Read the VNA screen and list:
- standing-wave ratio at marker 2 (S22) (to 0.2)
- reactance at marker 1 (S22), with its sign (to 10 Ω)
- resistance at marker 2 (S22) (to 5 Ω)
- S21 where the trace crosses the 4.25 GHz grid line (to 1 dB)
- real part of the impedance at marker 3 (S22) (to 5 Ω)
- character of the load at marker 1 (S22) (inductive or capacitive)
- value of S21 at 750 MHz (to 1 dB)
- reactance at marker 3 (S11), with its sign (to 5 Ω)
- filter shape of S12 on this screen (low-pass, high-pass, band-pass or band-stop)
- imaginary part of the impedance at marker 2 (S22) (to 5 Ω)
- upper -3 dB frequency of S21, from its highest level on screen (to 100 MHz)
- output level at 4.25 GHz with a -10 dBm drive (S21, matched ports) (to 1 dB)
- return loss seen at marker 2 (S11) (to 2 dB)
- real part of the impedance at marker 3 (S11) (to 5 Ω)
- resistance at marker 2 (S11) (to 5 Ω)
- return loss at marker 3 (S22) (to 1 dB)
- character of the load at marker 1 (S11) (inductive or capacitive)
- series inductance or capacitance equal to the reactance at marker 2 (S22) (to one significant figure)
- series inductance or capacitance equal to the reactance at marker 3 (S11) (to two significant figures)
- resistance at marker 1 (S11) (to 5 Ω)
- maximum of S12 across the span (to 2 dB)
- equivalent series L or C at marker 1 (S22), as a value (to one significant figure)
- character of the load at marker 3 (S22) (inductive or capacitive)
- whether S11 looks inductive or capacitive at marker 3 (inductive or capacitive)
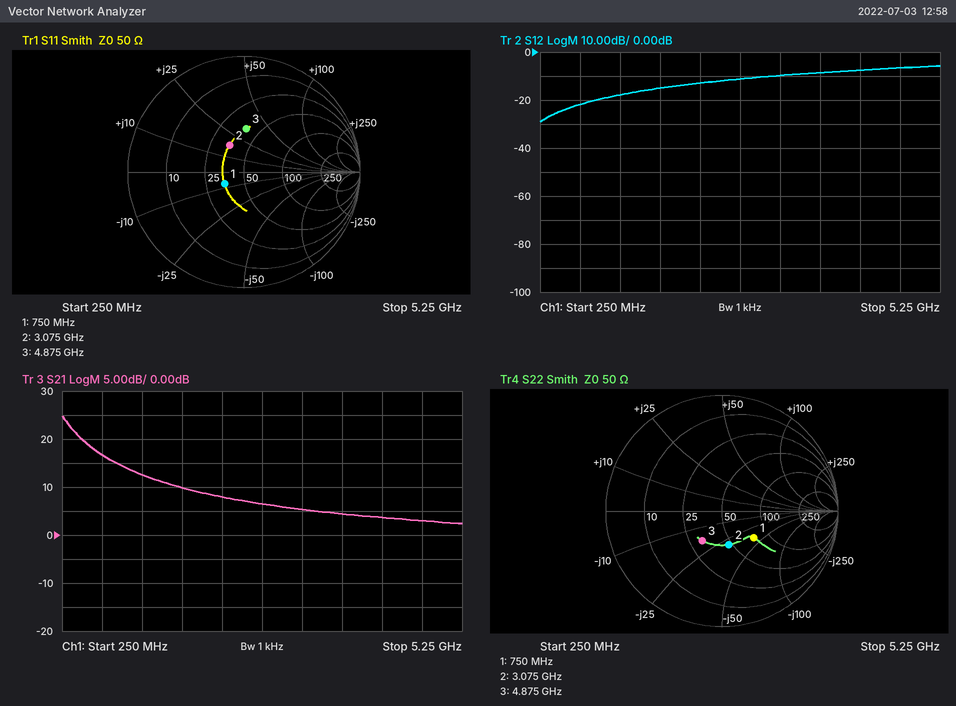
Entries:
1.8
-40 Ω
45 Ω
4 dB
30 Ω
capacitive
17 dB
+35 Ω
high-pass
-30 Ω
400 MHz
-6 dBm
12 dB
40 Ω
35 Ω
10 dB
capacitive
2 pF
1.1 nH
35 Ω
-6 dB
5 pF
capacitive
inductive
